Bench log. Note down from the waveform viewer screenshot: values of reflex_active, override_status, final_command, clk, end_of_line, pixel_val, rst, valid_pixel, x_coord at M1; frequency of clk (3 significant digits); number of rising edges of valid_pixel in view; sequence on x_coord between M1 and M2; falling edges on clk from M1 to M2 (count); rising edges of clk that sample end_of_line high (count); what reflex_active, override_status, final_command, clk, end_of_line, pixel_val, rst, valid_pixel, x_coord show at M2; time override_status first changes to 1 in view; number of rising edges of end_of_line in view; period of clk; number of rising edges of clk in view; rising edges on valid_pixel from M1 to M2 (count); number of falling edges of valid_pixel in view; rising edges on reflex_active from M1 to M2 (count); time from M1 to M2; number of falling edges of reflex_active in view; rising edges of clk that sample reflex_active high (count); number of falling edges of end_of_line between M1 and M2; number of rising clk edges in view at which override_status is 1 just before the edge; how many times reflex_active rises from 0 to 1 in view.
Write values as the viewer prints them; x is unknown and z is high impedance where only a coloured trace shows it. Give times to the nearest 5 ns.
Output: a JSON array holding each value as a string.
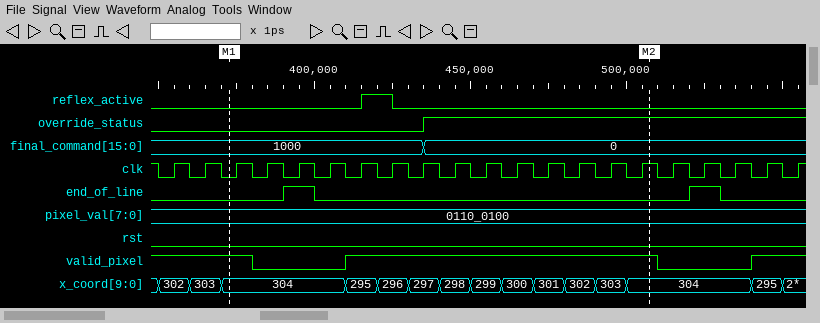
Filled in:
["reflex_active=0, override_status=0, final_command=1000, clk=0, end_of_line=0, pixel_val=0110_0100, rst=0, valid_pixel=1, x_coord=304", "100 MHz", "2", "304, 295, 296, 297, 298, 299, 300, 301, 302, 303, 304", "13", "2", "reflex_active=0, override_status=1, final_command=0, clk=1, end_of_line=0, pixel_val=0110_0100, rst=0, valid_pixel=1, x_coord=304", "435 ns", "2", "10 ns", "21", "1", "2", "1", "135 ns", "1", "1", "1", "12", "1"]
